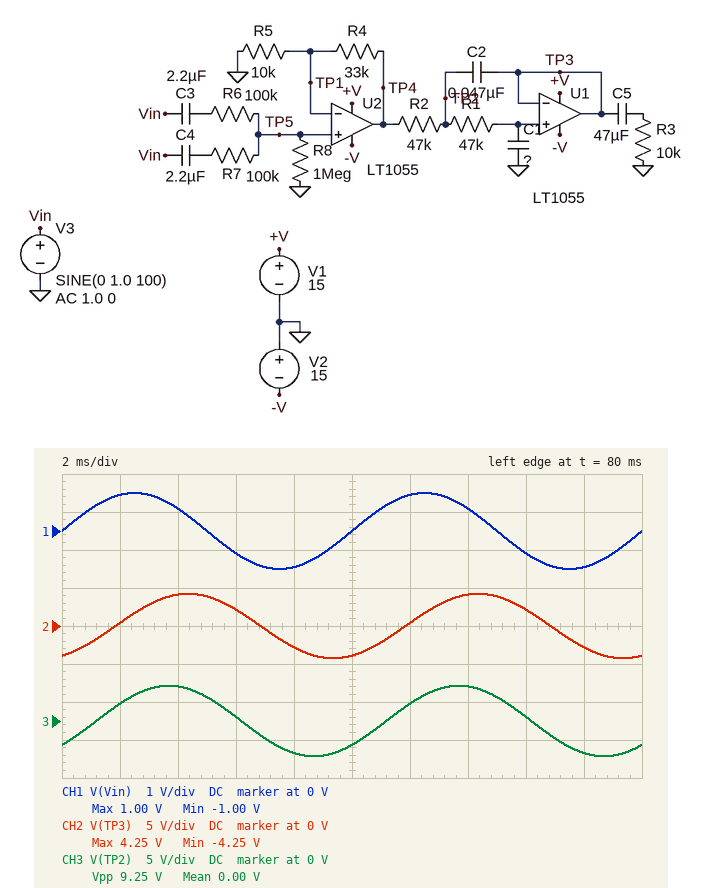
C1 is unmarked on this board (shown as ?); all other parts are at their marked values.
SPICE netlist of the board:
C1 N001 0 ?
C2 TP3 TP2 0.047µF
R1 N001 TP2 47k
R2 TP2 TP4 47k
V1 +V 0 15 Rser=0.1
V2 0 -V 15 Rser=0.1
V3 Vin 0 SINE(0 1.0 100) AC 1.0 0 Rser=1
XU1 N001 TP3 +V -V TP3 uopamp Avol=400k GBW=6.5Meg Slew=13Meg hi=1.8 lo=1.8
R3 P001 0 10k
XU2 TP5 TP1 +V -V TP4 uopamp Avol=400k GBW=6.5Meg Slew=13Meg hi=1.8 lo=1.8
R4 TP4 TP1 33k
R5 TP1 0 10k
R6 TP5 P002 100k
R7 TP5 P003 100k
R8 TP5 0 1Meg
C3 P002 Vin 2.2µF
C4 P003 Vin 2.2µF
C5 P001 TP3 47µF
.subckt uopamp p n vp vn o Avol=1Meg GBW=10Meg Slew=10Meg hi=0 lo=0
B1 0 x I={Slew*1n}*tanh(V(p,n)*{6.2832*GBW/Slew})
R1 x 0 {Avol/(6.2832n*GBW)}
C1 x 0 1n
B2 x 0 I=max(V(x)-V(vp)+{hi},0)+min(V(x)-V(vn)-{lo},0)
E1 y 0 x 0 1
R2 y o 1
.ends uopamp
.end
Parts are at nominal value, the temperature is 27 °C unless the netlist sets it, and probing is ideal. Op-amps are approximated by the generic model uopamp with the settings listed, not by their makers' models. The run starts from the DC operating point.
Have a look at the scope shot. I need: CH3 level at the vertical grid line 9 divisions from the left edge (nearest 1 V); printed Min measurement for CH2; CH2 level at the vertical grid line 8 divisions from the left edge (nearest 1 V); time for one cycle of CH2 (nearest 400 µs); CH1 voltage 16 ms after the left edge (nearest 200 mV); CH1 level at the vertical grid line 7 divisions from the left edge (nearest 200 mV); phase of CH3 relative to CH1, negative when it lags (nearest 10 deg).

-4 V
-4.25 V
2 V
10.0 ms
-600 mV
600 mV
-40 deg
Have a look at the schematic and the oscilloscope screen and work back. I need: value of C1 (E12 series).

15 nF
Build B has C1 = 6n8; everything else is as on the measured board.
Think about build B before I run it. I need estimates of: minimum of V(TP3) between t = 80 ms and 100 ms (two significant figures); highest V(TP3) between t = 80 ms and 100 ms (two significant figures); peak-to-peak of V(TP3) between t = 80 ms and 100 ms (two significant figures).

-5.0 V
5.0 V
9.9 V
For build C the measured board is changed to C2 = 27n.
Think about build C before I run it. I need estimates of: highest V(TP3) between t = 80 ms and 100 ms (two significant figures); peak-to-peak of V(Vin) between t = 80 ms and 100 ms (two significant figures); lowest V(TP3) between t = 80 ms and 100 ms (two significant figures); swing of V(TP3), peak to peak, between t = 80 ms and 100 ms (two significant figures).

3.7 V
2.0 V
-3.7 V
7.5 V
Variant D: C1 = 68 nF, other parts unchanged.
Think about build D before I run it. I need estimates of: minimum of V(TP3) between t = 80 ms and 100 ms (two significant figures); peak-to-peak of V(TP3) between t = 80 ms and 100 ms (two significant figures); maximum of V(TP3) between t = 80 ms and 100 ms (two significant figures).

-930 mV
1.9 V
930 mV
